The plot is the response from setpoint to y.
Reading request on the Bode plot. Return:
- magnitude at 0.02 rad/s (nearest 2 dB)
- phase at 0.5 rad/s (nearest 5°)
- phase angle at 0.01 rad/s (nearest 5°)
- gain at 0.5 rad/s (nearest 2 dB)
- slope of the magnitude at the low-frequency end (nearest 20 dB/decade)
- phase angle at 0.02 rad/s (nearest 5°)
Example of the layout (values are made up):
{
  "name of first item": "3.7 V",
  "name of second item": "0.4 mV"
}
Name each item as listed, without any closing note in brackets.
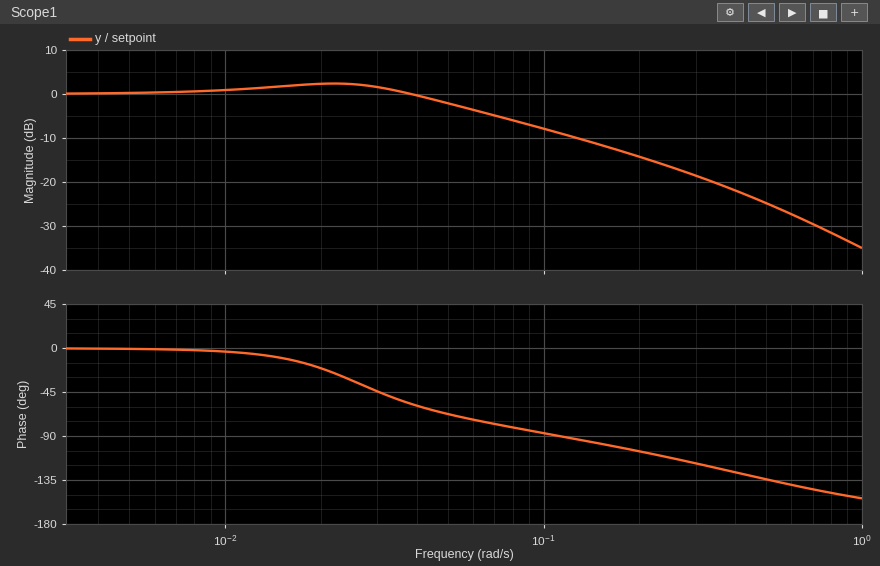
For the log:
{
  "magnitude at 0.02 rad/s": "2 dB",
  "phase at 0.5 rad/s": "-135°",
  "phase angle at 0.01 rad/s": "-5°",
  "gain at 0.5 rad/s": "-24 dB",
  "slope of the magnitude at the low-frequency end": "0 dB/decade",
  "phase angle at 0.02 rad/s": "-20°"
}
